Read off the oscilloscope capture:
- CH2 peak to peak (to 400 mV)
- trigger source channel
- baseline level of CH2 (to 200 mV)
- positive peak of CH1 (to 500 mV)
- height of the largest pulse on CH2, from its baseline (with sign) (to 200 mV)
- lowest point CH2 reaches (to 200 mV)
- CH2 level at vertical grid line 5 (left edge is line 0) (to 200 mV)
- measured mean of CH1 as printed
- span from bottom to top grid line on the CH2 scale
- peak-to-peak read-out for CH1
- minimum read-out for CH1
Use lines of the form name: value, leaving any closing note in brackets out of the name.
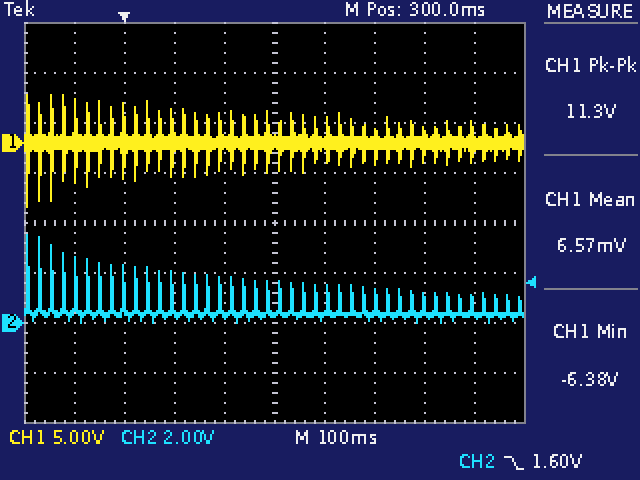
CH2 peak to peak: 3.6 V
trigger source channel: CH2
baseline level of CH2: 400 mV
positive peak of CH1: 5.0 V
height of the largest pulse on CH2, from its baseline (with sign): +3.2 V
lowest point CH2 reaches: 0.0 V
CH2 level at vertical grid line 5 (left edge is line 0): 400 mV
measured mean of CH1 as printed: 6.57 mV
span from bottom to top grid line on the CH2 scale: 16 V
peak-to-peak read-out for CH1: 11.3 V
minimum read-out for CH1: -6.38 V
